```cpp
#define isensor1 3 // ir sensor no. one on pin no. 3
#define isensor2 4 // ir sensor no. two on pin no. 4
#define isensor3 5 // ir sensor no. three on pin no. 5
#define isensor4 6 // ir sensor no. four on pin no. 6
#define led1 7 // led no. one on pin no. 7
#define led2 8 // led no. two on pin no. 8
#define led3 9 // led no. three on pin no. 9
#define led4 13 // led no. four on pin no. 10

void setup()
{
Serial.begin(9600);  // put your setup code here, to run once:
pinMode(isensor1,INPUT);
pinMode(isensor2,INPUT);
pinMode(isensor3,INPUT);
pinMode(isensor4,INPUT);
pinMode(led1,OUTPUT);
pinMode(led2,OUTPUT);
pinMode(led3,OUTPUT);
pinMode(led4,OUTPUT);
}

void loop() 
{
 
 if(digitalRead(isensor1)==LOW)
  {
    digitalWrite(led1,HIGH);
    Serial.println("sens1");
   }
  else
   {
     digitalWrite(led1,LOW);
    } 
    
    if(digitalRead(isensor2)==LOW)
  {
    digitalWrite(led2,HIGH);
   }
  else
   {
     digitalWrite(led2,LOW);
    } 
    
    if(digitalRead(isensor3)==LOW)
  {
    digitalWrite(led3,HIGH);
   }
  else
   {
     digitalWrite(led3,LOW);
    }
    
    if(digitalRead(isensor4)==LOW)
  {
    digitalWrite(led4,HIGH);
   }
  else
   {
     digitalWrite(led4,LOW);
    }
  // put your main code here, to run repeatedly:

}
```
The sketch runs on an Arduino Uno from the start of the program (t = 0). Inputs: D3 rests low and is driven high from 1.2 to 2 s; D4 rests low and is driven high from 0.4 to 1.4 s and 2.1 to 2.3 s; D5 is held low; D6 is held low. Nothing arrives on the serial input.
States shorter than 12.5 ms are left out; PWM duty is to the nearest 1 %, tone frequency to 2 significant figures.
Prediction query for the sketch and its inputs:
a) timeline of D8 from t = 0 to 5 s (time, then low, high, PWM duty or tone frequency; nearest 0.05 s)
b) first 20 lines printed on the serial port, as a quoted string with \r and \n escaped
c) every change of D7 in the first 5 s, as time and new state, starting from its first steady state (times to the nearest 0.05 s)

0 s high; 0.4 s low; 1.4 s high; 2.1 s low; 2.3 s high
"sens1\r\nsens1\r\nsens1\r\nsens1\r\nsens1\r\nsens1\r\nsens1\r\nsens1\r\nsens1\r\nsens1\r\nsens1\r\nsens1\r\nsens1\r\nsens1\r\nsens1\r\nsens1\r\nsens1\r\nsens1\r\nsens1\r\nsens1\r\n"
0 s high; 1.2 s low; 2 s high
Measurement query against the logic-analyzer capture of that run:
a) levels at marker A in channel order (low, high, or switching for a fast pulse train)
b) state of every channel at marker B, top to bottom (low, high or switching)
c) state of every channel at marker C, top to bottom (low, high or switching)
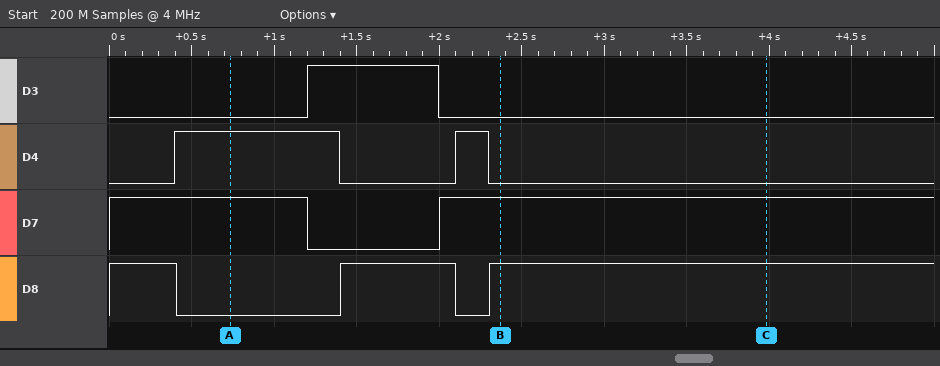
D3 low, D4 high, D7 high, D8 low
D3 low, D4 low, D7 high, D8 high
D3 low, D4 low, D7 high, D8 high
